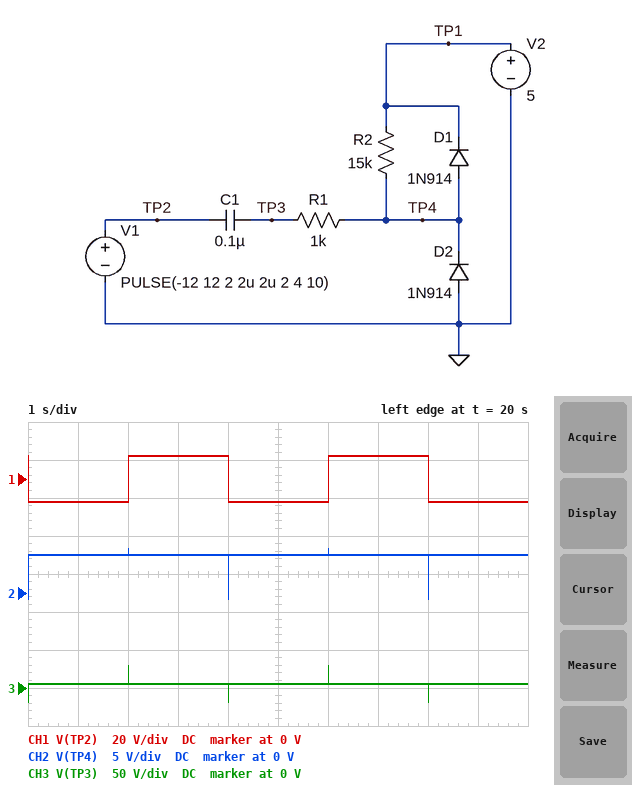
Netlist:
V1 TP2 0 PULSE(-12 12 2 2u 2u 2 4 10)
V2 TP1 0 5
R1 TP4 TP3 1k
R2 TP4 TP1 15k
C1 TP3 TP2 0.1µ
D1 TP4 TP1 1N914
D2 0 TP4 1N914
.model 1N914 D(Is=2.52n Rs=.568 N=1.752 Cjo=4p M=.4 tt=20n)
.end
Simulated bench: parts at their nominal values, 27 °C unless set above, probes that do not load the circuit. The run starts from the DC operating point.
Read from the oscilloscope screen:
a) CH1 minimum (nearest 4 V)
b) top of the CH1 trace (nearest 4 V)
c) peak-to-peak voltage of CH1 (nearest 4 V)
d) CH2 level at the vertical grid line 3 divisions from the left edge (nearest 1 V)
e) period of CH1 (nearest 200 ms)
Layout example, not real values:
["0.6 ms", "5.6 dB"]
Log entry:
["-12 V", "12 V", "24 V", "5 V", "4.0 s"]
